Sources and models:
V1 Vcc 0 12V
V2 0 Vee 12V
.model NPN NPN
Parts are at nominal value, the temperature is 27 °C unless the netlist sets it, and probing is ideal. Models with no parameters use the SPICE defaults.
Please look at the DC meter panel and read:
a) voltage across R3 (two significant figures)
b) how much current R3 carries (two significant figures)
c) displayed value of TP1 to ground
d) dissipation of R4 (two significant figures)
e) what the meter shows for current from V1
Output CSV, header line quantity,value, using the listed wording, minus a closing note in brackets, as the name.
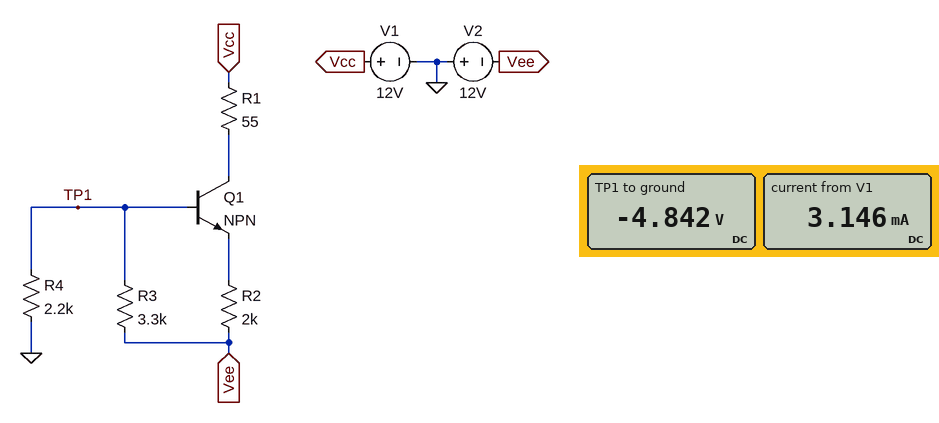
quantity,value
voltage across R3,7.2 V
how much current R3 carries,2.2 mA
displayed value of TP1 to ground,-4.842 V
dissipation of R4,11 mW
what the meter shows for current from V1,3.146 mA
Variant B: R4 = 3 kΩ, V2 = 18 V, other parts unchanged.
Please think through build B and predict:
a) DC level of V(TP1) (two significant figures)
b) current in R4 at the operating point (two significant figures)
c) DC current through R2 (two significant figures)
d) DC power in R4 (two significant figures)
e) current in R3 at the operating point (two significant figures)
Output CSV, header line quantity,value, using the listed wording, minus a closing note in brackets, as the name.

quantity,value
DC level of V(TP1),-8.6 V
current in R4 at the operating point,2.9 mA
DC current through R2,4.3 mA
DC power in R4,25 mW
current in R3 at the operating point,2.8 mA
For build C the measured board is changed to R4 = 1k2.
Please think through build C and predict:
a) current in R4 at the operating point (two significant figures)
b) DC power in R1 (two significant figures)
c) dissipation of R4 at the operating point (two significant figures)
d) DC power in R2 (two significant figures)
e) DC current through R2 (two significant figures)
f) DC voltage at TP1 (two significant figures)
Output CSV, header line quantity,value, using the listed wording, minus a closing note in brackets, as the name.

quantity,value
current in R4 at the operating point,2.7 mA
DC power in R1,850 µW
dissipation of R4 at the operating point,8.7 mW
DC power in R2,32 mW
DC current through R2,4.0 mA
DC voltage at TP1,-3.2 V
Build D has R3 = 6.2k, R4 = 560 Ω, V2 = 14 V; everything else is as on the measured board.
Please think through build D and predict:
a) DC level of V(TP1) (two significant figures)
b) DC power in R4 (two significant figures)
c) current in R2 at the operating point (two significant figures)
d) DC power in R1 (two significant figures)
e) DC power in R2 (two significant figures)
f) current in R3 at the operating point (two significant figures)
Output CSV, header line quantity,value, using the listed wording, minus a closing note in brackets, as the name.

quantity,value
DC level of V(TP1),-1.2 V
DC power in R4,2.5 mW
current in R2 at the operating point,6.0 mA
DC power in R1,1.9 mW
DC power in R2,72 mW
current in R3 at the operating point,2.1 mA
